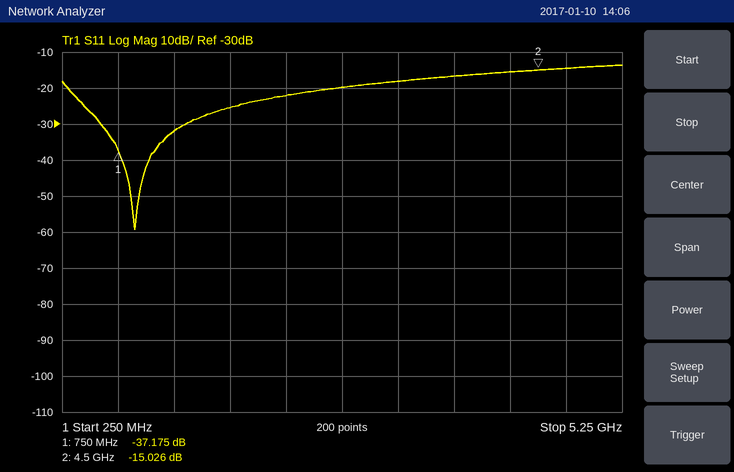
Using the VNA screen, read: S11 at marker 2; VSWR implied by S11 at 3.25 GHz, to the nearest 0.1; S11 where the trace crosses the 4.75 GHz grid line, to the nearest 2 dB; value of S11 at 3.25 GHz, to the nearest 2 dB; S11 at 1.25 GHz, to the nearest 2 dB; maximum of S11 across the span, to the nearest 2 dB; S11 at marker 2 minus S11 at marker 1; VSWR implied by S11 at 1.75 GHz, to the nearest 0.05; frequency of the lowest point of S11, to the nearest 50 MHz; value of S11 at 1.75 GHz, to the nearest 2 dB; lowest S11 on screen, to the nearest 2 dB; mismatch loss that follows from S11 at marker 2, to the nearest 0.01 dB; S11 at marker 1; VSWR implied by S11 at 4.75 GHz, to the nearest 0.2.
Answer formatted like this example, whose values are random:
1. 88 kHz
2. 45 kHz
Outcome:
1. -15.026 dB
2. 1.3
3. -14 dB
4. -18 dB
5. -32 dB
6. -14 dB
7. 22.149 dB
8. 1.10
9. 900 MHz
10. -26 dB
11. -60 dB
12. 0.14 dB
13. -37.175 dB
14. 1.4
